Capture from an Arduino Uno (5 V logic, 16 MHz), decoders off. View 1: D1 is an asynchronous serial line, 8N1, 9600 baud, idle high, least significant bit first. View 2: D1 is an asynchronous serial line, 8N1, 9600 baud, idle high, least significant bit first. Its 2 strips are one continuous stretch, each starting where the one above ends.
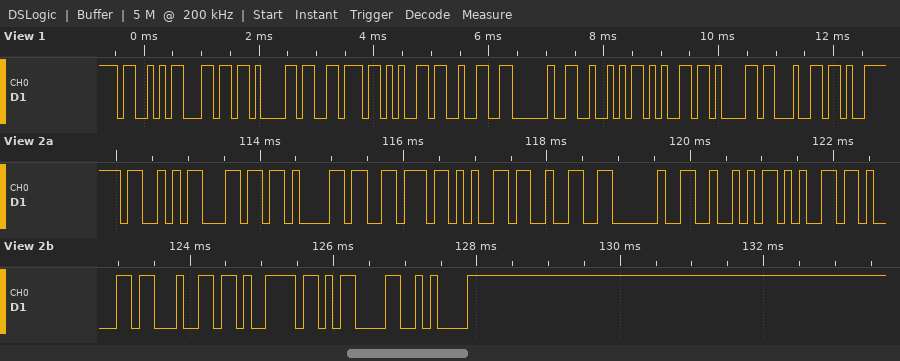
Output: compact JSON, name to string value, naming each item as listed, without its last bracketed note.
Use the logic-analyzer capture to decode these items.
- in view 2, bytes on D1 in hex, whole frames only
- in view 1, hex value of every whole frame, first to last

{"in view 2, bytes on D1 in hex, whole frames only": "53 6C 61 76 65 32 20 52 65 61 64 79 0D 0A", "in view 1, hex value of every whole frame, first to last": "0x53 0x6C 0x61 0x76 0x65 0x32 0x20 0x52 0x65 0x61 0x64"}
